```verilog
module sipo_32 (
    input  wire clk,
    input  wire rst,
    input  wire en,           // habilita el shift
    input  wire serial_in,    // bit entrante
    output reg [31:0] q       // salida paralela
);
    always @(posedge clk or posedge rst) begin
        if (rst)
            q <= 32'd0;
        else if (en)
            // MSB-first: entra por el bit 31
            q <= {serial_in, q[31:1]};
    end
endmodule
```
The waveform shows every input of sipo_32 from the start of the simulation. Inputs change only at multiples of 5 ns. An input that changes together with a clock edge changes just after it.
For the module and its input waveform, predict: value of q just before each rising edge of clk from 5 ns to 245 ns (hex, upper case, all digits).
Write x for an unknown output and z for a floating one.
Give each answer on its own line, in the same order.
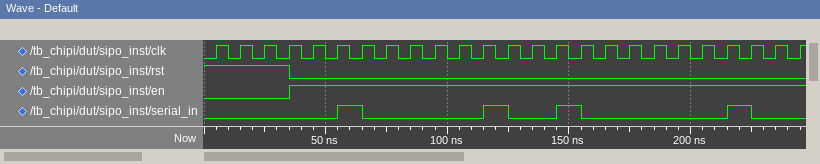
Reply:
00000000, 00000000, 00000000, 00000000, 00000000, 00000000, 00000000, 80000000, 40000000, 20000000, 10000000, 08000000, 04000000, 82000000, 41000000, 20800000, 90400000, 48200000, 24100000, 12080000, 09040000, 04820000, 02410000, 81208000, 40904000
